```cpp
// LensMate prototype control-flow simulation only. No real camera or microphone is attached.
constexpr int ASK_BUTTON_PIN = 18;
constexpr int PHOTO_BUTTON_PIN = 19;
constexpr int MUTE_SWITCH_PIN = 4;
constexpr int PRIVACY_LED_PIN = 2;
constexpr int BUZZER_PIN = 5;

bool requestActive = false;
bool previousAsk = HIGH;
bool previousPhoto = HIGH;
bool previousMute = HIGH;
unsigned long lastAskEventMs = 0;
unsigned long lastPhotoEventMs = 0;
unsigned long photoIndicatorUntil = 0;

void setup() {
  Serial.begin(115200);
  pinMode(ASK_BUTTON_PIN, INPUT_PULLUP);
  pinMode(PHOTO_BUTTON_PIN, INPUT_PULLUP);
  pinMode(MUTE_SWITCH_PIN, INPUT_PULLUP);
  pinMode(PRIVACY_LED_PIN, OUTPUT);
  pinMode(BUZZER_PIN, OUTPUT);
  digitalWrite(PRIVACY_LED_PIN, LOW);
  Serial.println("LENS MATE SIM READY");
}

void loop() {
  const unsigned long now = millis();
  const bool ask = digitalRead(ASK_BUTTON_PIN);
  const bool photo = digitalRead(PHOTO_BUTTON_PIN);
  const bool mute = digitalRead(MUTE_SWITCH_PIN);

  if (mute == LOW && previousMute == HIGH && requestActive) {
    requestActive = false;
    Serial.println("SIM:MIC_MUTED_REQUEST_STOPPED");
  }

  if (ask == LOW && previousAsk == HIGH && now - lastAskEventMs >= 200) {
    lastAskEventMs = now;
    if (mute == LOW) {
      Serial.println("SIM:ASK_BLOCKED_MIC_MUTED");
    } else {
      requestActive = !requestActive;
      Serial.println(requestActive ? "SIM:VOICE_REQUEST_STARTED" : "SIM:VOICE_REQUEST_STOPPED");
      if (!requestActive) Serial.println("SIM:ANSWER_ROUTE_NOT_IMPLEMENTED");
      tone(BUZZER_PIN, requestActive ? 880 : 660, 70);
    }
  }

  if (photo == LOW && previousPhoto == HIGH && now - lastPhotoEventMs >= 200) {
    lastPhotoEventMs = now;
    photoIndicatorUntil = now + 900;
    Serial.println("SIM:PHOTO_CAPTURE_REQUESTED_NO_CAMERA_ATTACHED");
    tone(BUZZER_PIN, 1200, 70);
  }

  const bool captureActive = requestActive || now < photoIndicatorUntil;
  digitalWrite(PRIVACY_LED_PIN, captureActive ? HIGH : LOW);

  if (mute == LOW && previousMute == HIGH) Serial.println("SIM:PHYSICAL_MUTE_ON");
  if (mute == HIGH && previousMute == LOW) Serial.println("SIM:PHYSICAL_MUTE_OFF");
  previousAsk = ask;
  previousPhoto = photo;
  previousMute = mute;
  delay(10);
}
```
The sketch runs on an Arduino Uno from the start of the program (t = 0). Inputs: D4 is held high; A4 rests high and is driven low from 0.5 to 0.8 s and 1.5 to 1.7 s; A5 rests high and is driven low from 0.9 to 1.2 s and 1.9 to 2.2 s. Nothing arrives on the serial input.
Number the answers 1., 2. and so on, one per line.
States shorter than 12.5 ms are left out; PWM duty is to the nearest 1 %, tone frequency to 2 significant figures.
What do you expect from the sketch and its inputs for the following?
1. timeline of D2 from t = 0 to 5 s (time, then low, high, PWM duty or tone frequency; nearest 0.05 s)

1. 0 s low; 0.5 s high; 1.8 s low; 1.9 s high; 2.8 s low
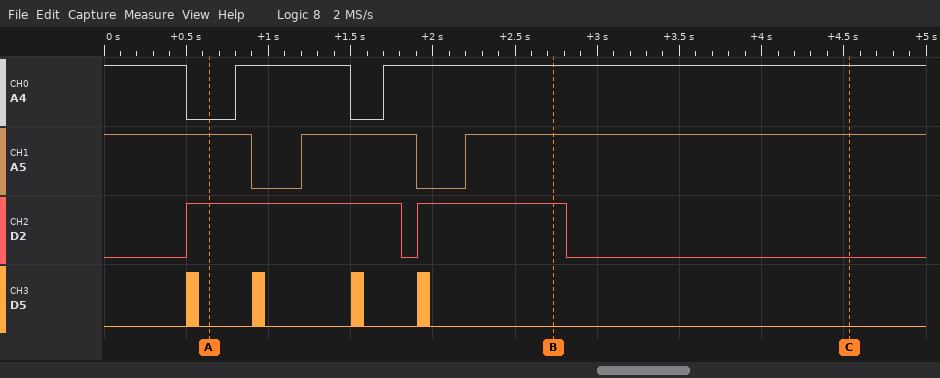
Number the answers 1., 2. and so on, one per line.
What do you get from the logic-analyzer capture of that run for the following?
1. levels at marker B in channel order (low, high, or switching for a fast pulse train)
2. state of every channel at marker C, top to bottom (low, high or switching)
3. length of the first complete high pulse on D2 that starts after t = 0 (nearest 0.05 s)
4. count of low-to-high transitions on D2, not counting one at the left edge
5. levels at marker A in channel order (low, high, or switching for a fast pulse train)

1. A4 high, A5 high, D2 high, D5 low
2. A4 high, A5 high, D2 low, D5 low
3. 1.30 s
4. 2
5. A4 low, A5 high, D2 high, D5 low
